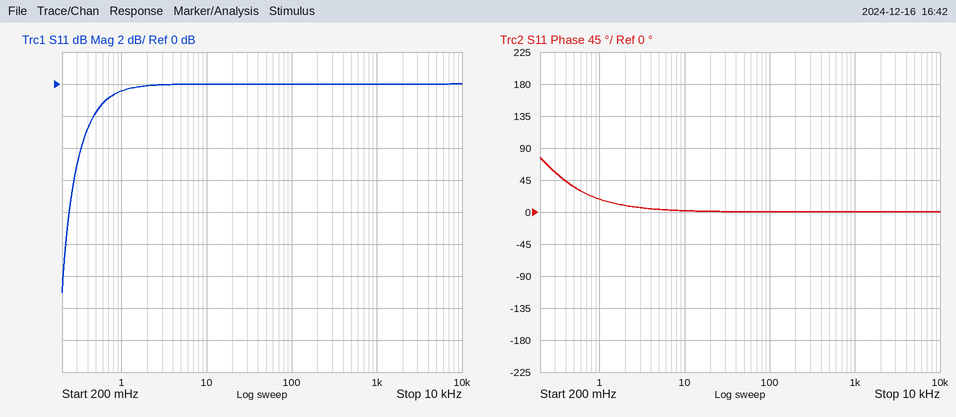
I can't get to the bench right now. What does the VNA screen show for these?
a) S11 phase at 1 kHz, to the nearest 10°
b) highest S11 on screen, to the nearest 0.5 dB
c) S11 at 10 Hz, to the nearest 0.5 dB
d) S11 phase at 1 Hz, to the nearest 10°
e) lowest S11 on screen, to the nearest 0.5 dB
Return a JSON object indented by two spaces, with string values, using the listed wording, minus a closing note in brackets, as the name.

{
  "S11 phase at 1 kHz, to the nearest 10°": "0°",
  "highest S11 on screen, to the nearest 0.5 dB": "0.0 dB",
  "S11 at 10 Hz, to the nearest 0.5 dB": "0.0 dB",
  "S11 phase at 1 Hz, to the nearest 10°": "20°",
  "lowest S11 on screen, to the nearest 0.5 dB": "-13.0 dB"
}
